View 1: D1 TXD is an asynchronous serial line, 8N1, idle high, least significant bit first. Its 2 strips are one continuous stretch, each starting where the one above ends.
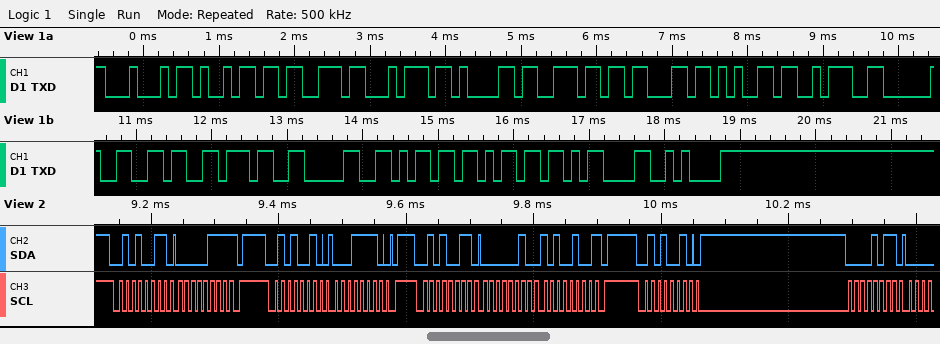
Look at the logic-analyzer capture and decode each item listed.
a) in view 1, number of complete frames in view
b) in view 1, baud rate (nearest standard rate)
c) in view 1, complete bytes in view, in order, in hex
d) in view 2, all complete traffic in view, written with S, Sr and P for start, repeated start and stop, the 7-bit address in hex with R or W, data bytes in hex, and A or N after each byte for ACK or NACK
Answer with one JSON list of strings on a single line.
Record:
["17", "9600 baud", "0x44 0x69 0x73 0x74 0x61 0x6E 0x63 0x65 0x3A 0x20 0x36 0x37 0x30 0x6D 0x6D 0x0D 0x0A", "S 29R A 07 N P S 29W A 1E A P S 29R A 02 A A4 N P S 29W A 0B A"]
